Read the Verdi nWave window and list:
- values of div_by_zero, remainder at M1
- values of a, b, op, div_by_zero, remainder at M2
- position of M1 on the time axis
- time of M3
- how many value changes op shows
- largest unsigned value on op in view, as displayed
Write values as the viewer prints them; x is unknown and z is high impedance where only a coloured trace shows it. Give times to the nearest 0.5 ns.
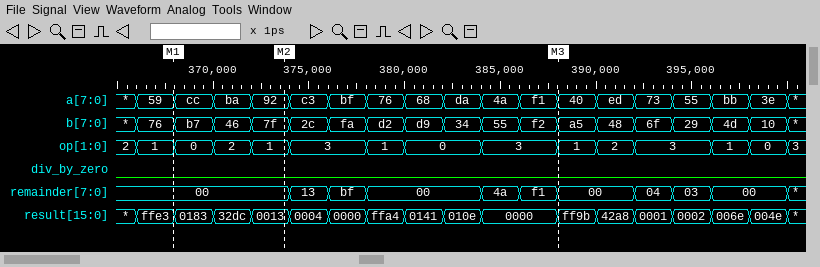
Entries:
div_by_zero=0, remainder=00
a=92, b=7f, op=1, div_by_zero=0, remainder=00
368 ns
388 ns
14
3
